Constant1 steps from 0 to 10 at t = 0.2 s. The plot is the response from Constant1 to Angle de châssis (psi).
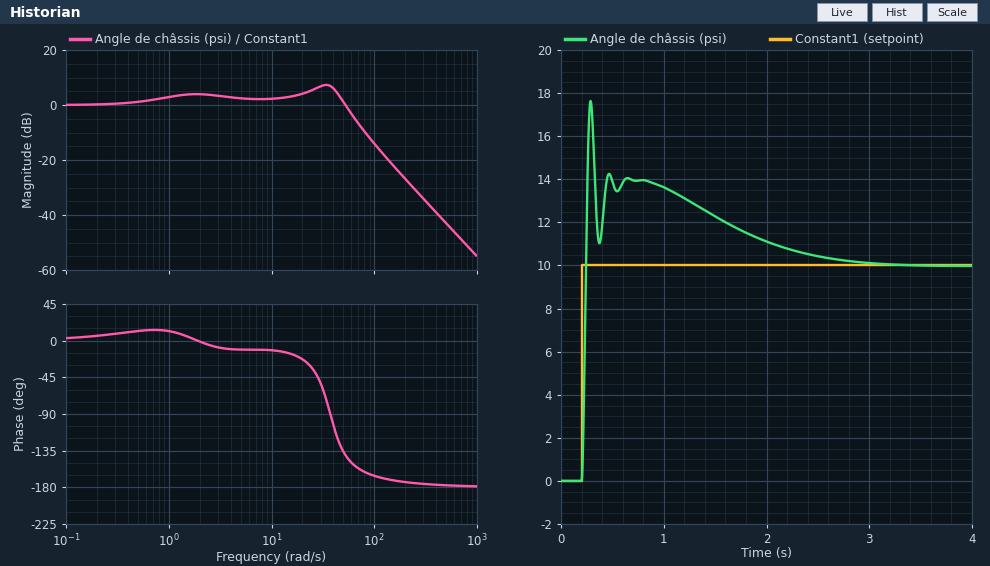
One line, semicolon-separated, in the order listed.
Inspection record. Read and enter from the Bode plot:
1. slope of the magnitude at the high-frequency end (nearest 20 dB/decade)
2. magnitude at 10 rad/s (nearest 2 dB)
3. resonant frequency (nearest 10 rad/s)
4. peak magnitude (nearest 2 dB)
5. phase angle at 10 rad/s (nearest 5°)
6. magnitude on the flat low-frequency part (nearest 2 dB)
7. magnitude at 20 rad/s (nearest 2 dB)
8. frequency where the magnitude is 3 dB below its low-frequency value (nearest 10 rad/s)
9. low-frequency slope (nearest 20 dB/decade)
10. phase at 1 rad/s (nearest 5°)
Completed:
-40 dB/decade; 2 dB; 30 rad/s; 8 dB; -10°; 0 dB; 4 dB; 60 rad/s; 0 dB/decade; 10°
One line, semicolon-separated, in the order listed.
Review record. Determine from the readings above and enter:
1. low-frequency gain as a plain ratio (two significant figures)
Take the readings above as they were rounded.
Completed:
1.0
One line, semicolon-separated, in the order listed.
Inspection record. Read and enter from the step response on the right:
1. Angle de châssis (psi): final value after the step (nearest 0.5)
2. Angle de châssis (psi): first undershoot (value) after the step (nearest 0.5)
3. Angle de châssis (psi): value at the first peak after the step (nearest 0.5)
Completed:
10.0; 11.0; 17.5
